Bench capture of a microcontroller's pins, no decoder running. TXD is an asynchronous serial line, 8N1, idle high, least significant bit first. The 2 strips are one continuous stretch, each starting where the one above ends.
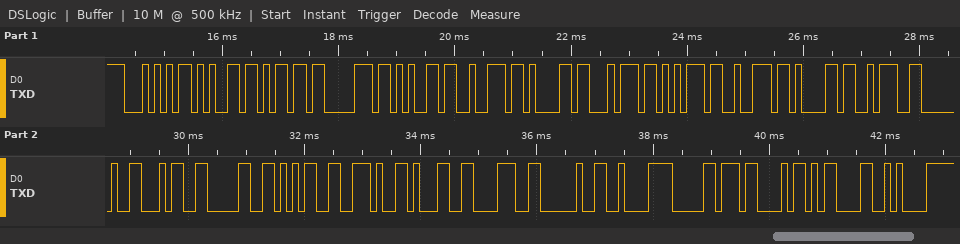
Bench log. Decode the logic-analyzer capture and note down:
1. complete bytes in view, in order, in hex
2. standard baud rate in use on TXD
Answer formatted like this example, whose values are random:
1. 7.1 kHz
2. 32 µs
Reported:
1. 54 65 6D 70 65 72 61 74 75 72 61 3A 20 34 30 35 2E 31 38 20 C2 B0 43 0D 0A
2. 9600 baud
